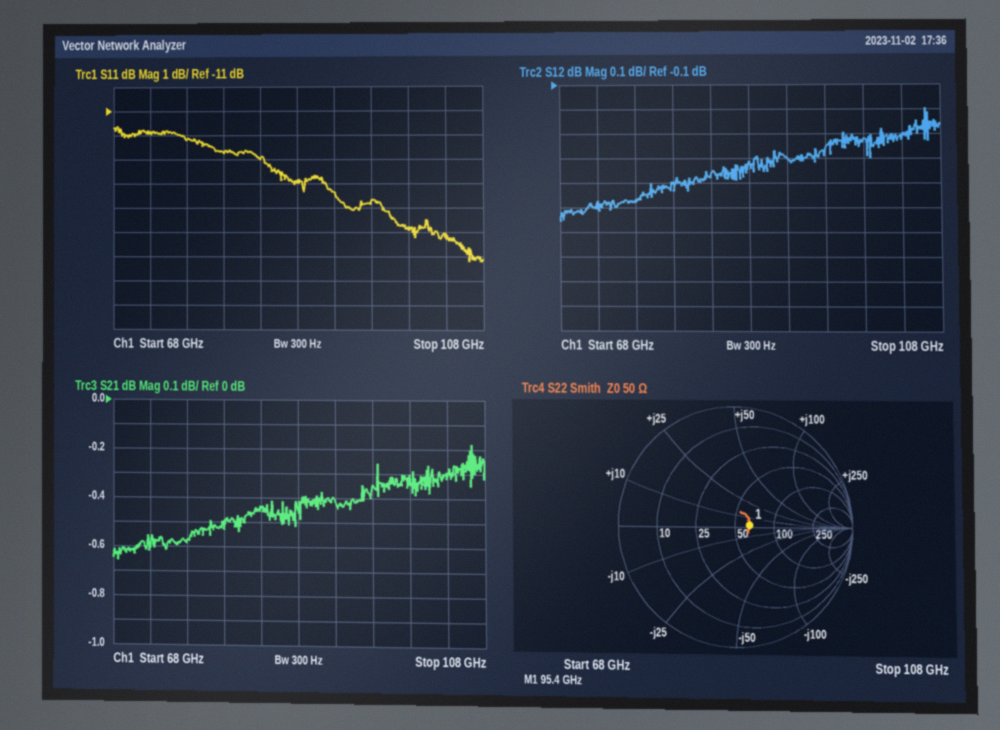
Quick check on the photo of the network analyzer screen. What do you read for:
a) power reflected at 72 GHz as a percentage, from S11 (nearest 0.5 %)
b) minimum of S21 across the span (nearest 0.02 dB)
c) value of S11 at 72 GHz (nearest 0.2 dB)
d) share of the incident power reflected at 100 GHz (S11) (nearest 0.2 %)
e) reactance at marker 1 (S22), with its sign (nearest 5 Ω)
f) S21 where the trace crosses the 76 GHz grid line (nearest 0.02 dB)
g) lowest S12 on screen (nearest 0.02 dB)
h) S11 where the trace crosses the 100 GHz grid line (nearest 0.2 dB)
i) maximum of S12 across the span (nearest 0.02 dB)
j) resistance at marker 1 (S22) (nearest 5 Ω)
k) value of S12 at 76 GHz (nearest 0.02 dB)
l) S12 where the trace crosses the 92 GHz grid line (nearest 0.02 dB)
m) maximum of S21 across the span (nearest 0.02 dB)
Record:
6.5 %
-0.66 dB
-11.8 dB
2.6 %
0 Ω
-0.58 dB
-0.66 dB
-15.8 dB
-0.20 dB
65 Ω
-0.58 dB
-0.40 dB
-0.18 dB
